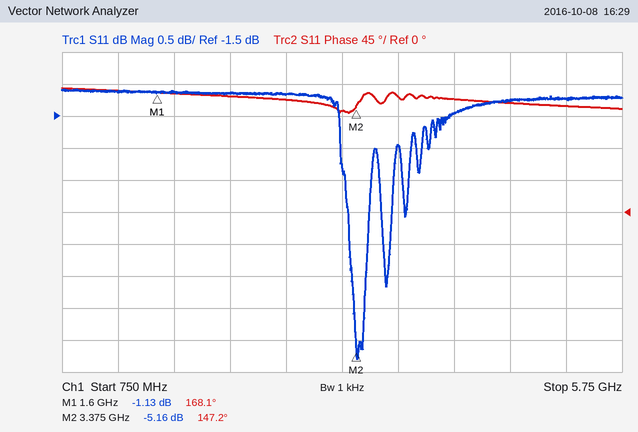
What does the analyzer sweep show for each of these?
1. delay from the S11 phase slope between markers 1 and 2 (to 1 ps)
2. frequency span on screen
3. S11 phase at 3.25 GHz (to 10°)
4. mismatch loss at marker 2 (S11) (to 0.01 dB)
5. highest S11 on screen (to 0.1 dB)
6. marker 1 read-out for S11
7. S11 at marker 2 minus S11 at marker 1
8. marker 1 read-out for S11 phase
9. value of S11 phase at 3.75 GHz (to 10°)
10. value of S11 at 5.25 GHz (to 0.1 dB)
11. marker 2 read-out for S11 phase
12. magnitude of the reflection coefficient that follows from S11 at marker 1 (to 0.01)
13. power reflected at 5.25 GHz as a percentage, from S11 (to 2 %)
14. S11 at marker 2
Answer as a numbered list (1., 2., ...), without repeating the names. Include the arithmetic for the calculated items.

1. −(147.2° − (168.1°))/(360° × 1.775 GHz) ≈ 33 ps
2. 5 GHz
3. 140°
4. −10 log10(1 − 10^(-5.16/10)) ≈ 1.58 dB
5. -1.1 dB
6. -1.13 dB
7. -5.16 − (-1.13) = -4.03 dB
8. 168.1°
9. 160°
10. -1.2 dB
11. 147.2°
12. 10^(-1.13/20) ≈ 0.88
13. 10^(-1.2/10) ≈ 76 %
14. -5.16 dB
